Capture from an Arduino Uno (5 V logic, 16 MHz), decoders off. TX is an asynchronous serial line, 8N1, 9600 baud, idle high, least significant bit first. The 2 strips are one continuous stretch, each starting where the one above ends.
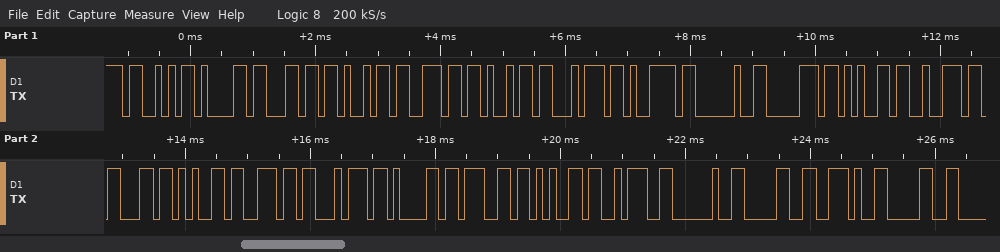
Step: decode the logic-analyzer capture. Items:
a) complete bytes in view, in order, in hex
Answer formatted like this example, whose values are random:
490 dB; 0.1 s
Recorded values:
53 61 6C 69 6E 69 74 79 20 70 65 72 63 65 6E 74 61 67 65 3A 20 30 2E 30
